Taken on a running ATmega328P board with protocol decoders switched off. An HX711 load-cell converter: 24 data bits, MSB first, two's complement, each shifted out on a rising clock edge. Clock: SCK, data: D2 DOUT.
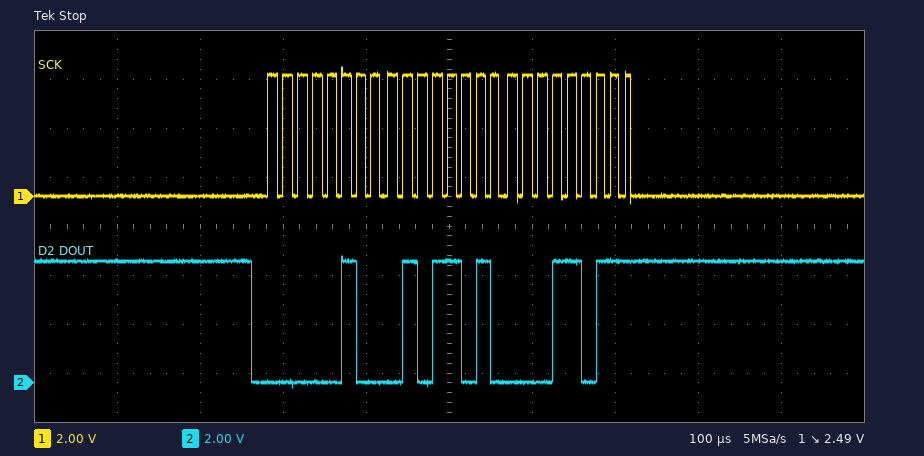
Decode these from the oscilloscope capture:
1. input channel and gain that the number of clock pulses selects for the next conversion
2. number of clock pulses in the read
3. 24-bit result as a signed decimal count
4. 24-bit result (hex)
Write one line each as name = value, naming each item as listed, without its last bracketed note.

input channel and gain that the number of clock pulses selects for the next conversion = channel A, gain 128
number of clock pulses in the read = 25
24-bit result as a signed decimal count = 285211
24-bit result = 0x045A1B
